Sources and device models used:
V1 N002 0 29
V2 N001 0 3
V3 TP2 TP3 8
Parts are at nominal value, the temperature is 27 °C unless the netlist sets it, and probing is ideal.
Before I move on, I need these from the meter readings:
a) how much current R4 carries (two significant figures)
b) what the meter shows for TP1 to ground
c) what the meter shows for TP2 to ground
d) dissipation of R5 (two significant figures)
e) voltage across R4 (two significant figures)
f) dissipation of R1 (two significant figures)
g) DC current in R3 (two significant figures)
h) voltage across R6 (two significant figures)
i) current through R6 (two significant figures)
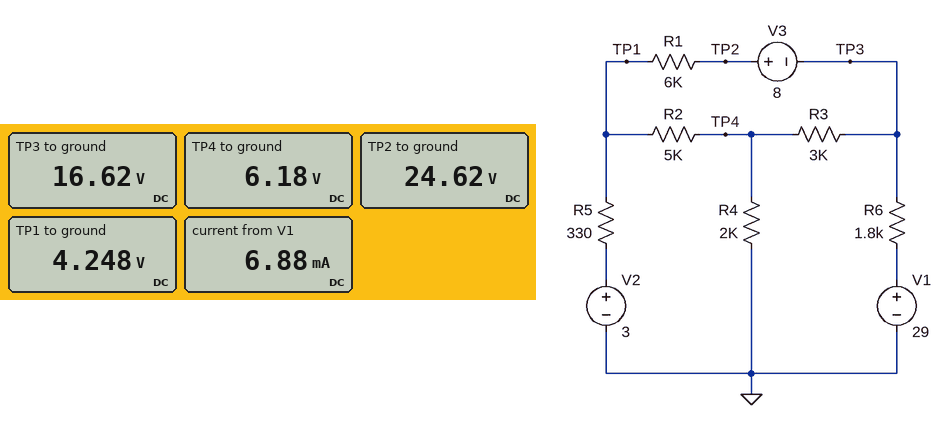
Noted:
3.1 mA
4.248 V
24.62 V
4.7 mW
6.2 V
69 mW
3.5 mA
12 V
6.9 mA
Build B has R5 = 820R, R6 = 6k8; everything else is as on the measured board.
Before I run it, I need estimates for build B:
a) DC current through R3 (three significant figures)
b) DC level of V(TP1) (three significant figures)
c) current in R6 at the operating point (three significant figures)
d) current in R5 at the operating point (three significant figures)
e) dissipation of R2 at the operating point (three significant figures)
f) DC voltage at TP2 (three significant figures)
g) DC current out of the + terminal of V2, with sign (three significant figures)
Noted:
1.37 mA
4.31 V
3.19 mA
1.60 mA
255 µW
15.3 V
-1.60 mA
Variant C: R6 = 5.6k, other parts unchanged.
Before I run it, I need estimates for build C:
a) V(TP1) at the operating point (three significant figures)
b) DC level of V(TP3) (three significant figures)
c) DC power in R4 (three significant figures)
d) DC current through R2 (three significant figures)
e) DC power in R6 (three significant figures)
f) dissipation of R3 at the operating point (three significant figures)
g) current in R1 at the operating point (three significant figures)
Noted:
3.67 V
8.22 V
5.65 mW
61.6 µA
77.1 mW
7.87 mW
2.09 mA
